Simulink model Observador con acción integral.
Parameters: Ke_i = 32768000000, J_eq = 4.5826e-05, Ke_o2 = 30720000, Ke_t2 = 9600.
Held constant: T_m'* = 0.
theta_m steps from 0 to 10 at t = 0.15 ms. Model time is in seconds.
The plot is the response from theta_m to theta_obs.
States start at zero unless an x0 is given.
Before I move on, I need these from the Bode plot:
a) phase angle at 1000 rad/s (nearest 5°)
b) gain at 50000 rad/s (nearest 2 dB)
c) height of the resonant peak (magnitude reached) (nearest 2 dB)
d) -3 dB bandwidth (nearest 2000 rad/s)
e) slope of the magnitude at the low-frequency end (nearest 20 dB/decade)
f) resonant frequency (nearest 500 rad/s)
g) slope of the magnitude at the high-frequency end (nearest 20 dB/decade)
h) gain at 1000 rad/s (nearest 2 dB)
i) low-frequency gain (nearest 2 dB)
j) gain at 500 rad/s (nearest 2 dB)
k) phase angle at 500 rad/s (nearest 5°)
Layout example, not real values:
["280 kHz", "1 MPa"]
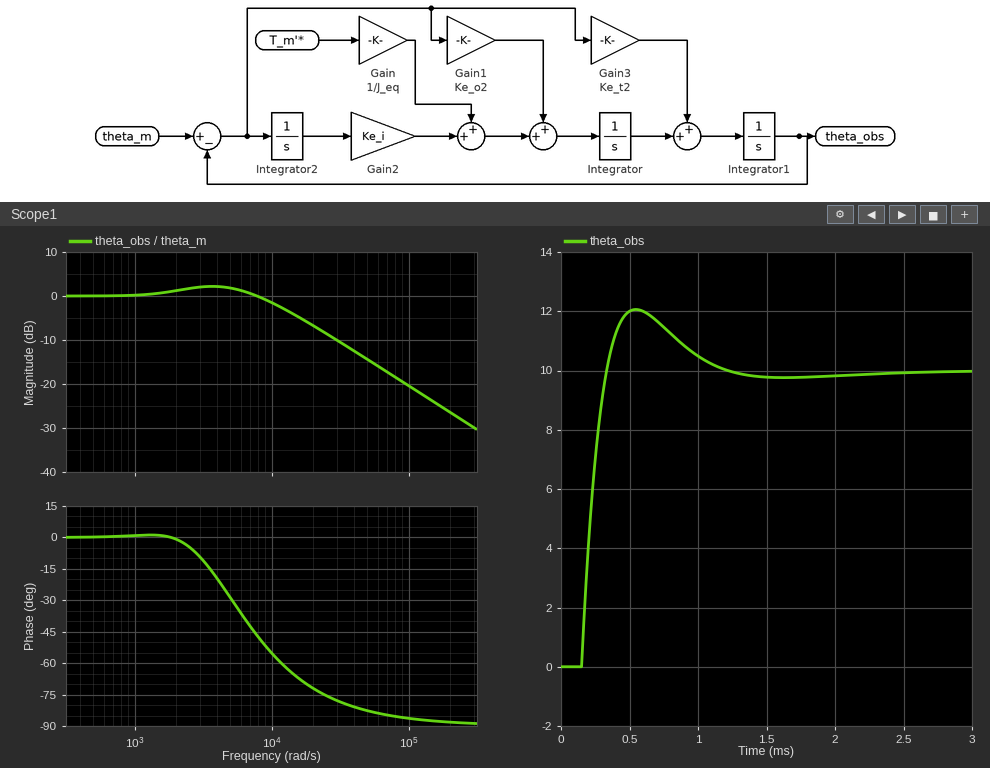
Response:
["0°", "-14 dB", "2 dB", "12000 rad/s", "0 dB/decade", "3500 rad/s", "-20 dB/decade", "0 dB", "0 dB", "0 dB", "0°"]
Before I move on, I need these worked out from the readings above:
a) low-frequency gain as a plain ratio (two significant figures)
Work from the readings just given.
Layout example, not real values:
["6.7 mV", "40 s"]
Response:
["1.0"]
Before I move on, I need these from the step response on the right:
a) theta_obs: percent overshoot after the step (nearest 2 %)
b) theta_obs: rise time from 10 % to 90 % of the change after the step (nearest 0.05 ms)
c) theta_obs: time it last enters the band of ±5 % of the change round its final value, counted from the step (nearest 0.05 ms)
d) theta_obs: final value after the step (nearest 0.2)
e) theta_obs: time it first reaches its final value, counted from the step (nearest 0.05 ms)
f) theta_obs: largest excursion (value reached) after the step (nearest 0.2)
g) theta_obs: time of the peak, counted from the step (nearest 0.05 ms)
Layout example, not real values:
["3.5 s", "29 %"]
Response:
["20 %", "0.15 ms", "0.85 ms", "10.0", "0.20 ms", "12.0", "0.40 ms"]
